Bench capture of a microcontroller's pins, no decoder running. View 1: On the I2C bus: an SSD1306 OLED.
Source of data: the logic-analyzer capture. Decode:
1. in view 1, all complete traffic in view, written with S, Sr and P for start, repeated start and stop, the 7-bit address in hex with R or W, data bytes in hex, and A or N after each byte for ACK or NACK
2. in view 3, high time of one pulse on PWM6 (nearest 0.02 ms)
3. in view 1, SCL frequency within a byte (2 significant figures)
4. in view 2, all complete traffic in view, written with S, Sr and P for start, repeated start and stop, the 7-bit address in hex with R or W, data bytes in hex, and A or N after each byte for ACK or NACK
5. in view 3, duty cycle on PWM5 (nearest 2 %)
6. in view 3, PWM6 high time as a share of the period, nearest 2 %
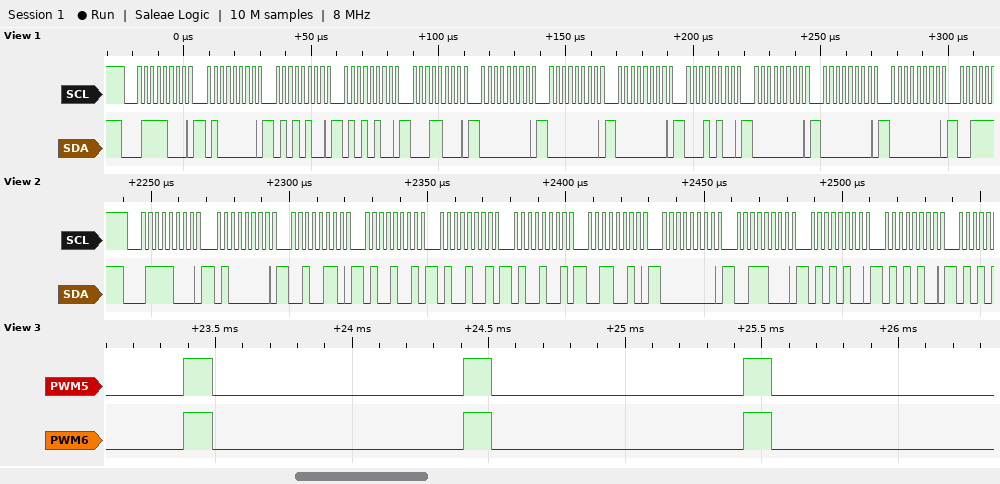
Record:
S 3CW A 40 A 54 A 54 A 18 A 00 A 00 A 00 A 14 A 00 A 00 A 00 A
0.10 ms
400 kHz
S 3CW A 40 A 26 A 49 A 49 A 49 A 32 A 00 A 38 A 54 A 54 A
10 %
10 %
